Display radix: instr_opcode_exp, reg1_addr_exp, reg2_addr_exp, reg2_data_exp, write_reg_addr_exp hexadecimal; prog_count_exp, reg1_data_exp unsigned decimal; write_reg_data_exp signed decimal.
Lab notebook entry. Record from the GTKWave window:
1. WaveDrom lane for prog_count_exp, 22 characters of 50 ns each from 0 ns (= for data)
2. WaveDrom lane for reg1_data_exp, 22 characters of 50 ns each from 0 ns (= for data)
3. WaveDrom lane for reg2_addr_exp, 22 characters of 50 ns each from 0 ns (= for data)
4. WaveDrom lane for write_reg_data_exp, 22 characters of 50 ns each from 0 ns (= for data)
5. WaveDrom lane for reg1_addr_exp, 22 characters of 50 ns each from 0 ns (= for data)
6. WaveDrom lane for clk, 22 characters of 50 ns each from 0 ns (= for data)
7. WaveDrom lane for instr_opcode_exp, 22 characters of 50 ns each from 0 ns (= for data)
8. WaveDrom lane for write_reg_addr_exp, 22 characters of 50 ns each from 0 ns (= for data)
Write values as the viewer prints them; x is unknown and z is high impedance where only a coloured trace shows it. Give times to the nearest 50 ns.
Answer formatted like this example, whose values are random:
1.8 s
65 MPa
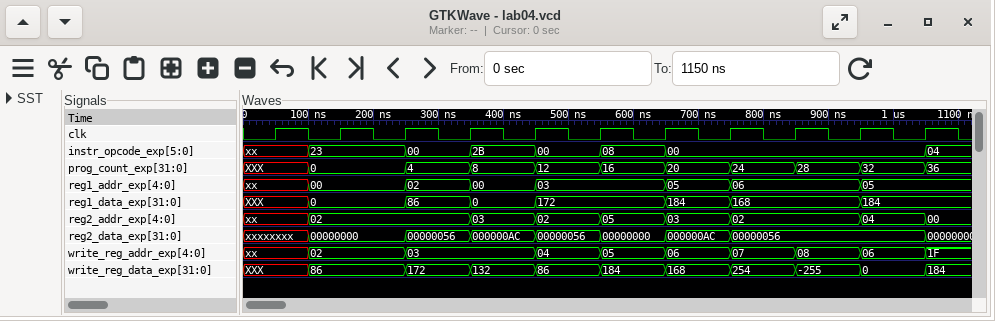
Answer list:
{name: 'prog_count_exp', wave: 'x.=..=.=.=.=.=.=.=.=.=', data: '0 4 8 12 16 20 24 28 32 36'}
{name: 'reg1_data_exp', wave: 'x.=..=.=.=...=.=...=..', data: '0 86 0 172 184 168 184'}
{name: 'reg2_addr_exp', wave: 'x.=....=.=.=.=.=...=.=', data: '02 03 02 05 03 02 04 00'}
{name: 'write_reg_data_exp', wave: 'x.=..=.=.=.=.=.=.=.=.=', data: '86 172 132 86 184 168 254 -255 0 184'}
{name: 'reg1_addr_exp', wave: 'x.=..=.=.=...=.=...=..', data: '00 02 00 03 05 06 05'}
{name: 'clk', wave: '0101010101010101010101'}
{name: 'instr_opcode_exp', wave: 'x.=..=.=.=.=.=.......=', data: '23 00 2B 00 08 00 04'}
{name: 'write_reg_addr_exp', wave: 'x.=..=...=.=.=.=.=.=.=', data: '02 03 04 05 06 07 08 06 1F'}
